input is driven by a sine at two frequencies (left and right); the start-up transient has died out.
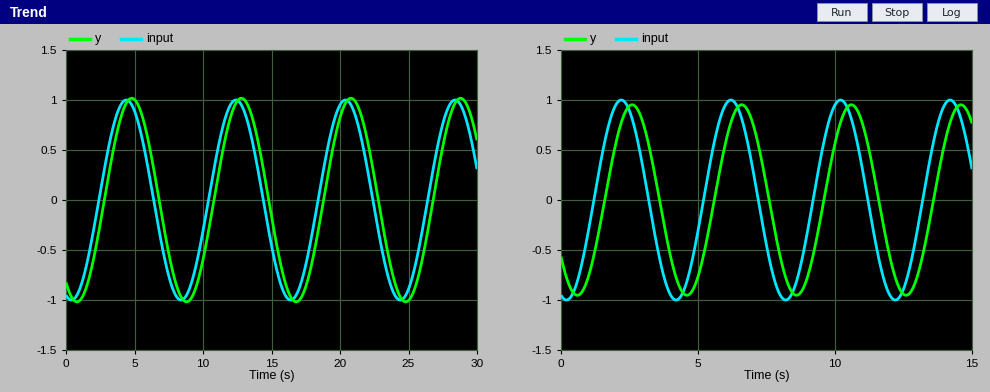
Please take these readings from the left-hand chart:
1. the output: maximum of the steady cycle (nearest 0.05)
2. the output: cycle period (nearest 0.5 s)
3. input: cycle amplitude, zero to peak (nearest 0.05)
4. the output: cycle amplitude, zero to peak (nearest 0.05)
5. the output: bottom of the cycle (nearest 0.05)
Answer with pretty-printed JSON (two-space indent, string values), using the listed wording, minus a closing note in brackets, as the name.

{
  "the output: maximum of the steady cycle": "1.00",
  "the output: cycle period": "8.0 s",
  "input: cycle amplitude, zero to peak": "1.00",
  "the output: cycle amplitude, zero to peak": "1.00",
  "the output: bottom of the cycle": "-1.00"
}
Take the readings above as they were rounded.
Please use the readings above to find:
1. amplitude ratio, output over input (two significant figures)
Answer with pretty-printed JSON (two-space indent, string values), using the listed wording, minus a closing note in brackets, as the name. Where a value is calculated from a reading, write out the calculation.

{
  "amplitude ratio, output over input": "1 / 1 = 1.0"
}
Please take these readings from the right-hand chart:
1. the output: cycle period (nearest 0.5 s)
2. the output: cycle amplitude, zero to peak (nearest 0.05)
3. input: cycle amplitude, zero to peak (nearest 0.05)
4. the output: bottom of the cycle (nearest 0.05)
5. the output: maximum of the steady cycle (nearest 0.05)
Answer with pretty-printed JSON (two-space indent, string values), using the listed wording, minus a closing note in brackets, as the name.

{
  "the output: cycle period": "4.0 s",
  "the output: cycle amplitude, zero to peak": "0.95",
  "input: cycle amplitude, zero to peak": "1.00",
  "the output: bottom of the cycle": "-0.95",
  "the output: maximum of the steady cycle": "0.95"
}
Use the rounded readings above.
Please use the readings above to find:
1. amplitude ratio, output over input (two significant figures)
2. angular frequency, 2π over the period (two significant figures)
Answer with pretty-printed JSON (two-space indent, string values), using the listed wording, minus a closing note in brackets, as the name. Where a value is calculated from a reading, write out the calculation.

{
  "amplitude ratio, output over input": "0.95 / 1 = 0.95",
  "angular frequency, 2π over the period": "2π / 4 = 1.6 rad/s"
}
